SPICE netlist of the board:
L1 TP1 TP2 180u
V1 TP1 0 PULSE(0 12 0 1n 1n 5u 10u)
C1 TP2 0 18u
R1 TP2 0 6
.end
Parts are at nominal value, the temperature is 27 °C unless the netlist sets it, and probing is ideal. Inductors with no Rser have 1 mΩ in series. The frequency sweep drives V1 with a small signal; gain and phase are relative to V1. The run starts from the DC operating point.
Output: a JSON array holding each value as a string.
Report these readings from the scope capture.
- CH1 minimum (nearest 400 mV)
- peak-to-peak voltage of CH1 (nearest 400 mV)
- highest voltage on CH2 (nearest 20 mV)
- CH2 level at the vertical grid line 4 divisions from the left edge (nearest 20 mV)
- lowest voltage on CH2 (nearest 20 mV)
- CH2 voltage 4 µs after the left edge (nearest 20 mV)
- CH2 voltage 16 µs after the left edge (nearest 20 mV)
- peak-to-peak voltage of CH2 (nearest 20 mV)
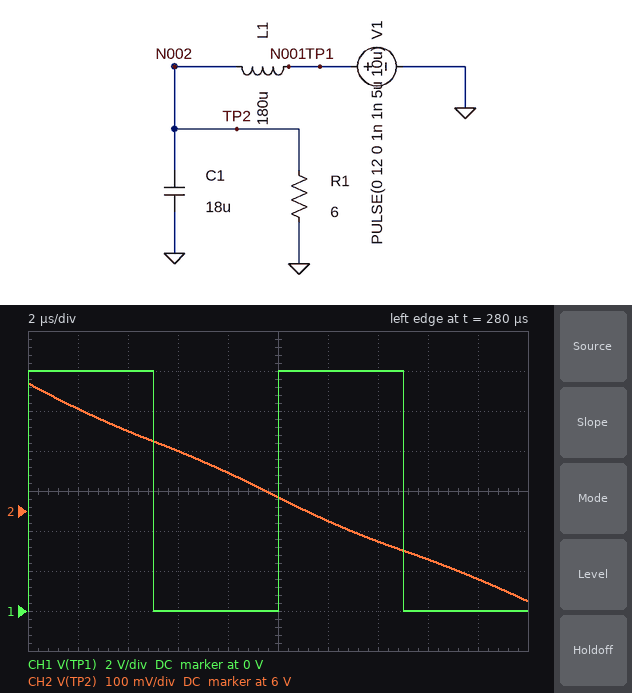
["0 V", "12.0 V", "6.32 V", "6.10 V", "5.78 V", "6.20 V", "5.88 V", "540 mV"]
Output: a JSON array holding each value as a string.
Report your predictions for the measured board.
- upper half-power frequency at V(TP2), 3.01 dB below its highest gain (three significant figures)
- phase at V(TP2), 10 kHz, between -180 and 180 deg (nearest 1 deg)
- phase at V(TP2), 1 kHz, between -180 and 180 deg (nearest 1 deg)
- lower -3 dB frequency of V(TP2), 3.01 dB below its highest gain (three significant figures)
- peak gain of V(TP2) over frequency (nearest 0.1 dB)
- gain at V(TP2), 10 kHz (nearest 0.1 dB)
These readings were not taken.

["3.27 kHz", "-171 deg", "-12 deg", "1.66 kHz", "5.9 dB", "-21.5 dB"]
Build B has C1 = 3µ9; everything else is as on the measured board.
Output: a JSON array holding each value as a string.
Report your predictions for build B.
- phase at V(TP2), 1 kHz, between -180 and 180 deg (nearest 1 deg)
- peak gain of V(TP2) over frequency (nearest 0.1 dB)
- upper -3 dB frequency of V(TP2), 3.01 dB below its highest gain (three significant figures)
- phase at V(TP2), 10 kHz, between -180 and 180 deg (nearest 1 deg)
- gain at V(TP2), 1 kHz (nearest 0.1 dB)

["-11 deg", "0.6 dB", "6.83 kHz", "-133 deg", "0.1 dB"]
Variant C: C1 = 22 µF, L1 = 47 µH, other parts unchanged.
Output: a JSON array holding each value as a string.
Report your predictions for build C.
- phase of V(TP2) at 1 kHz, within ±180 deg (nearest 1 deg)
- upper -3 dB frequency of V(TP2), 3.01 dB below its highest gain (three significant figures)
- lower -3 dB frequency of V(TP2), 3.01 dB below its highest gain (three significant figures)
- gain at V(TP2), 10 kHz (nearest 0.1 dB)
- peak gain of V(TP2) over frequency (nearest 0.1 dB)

["-3 deg", "5.45 kHz", "4.22 kHz", "-9.9 dB", "12.3 dB"]
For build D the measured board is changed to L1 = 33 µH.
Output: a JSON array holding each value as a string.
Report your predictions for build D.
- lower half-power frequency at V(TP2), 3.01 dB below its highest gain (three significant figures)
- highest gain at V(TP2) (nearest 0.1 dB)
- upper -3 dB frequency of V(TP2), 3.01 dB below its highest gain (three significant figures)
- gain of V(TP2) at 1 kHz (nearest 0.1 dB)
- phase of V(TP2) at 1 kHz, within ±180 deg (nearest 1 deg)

["5.65 kHz", "13.0 dB", "7.15 kHz", "0.2 dB", "-2 deg"]
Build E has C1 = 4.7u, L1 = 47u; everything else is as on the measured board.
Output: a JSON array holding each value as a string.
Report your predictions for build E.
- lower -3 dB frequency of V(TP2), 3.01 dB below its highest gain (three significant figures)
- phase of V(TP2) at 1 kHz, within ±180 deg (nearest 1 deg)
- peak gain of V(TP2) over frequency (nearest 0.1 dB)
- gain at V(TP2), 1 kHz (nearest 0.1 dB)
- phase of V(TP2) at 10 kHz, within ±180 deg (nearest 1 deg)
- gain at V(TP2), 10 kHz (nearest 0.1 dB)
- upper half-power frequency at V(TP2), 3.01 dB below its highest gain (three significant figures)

["6.36 kHz", "-3 deg", "5.9 dB", "0.1 dB", "-75 deg", "5.9 dB", "12.5 kHz"]
